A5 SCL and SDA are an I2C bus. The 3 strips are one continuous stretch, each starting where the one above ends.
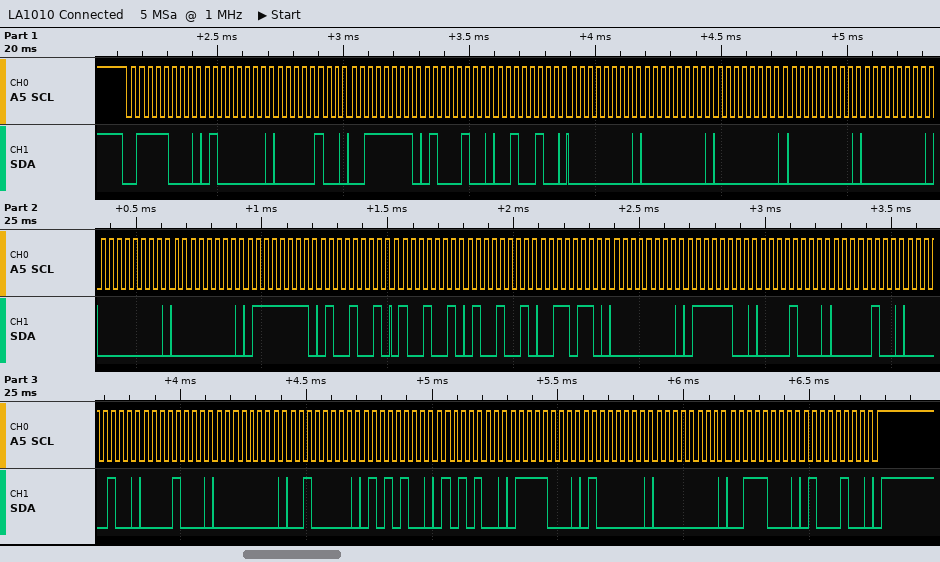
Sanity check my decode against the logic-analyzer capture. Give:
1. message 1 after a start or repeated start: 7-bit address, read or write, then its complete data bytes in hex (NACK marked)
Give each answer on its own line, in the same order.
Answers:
0x3C write: 40 04 3F 44 24 00 00 00 00 00 00 00 7F 49 49 49 36 00 7C 08 04 04 08 00 20 54 54 78 40 00 38 44
